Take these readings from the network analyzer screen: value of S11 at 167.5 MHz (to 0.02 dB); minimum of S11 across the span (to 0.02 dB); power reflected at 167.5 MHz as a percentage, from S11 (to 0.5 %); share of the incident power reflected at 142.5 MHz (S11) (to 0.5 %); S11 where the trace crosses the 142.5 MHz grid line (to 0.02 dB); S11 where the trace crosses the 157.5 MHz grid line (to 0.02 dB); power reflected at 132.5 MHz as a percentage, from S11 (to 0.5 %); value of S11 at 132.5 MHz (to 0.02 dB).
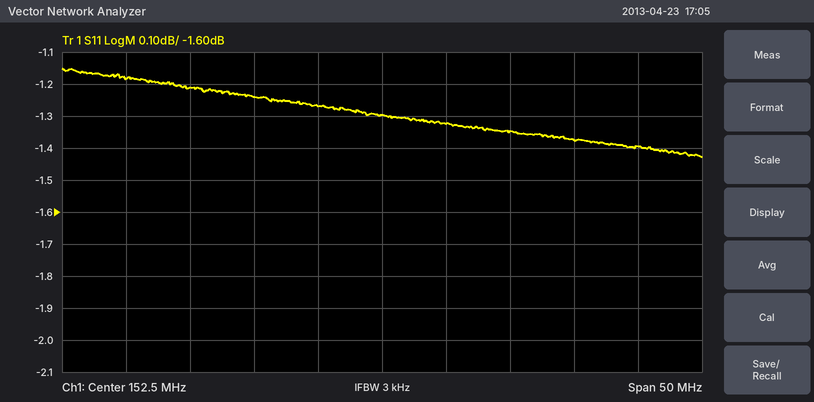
-1.38 dB
-1.42 dB
73.0 %
75.0 %
-1.24 dB
-1.32 dB
76.0 %
-1.18 dB
